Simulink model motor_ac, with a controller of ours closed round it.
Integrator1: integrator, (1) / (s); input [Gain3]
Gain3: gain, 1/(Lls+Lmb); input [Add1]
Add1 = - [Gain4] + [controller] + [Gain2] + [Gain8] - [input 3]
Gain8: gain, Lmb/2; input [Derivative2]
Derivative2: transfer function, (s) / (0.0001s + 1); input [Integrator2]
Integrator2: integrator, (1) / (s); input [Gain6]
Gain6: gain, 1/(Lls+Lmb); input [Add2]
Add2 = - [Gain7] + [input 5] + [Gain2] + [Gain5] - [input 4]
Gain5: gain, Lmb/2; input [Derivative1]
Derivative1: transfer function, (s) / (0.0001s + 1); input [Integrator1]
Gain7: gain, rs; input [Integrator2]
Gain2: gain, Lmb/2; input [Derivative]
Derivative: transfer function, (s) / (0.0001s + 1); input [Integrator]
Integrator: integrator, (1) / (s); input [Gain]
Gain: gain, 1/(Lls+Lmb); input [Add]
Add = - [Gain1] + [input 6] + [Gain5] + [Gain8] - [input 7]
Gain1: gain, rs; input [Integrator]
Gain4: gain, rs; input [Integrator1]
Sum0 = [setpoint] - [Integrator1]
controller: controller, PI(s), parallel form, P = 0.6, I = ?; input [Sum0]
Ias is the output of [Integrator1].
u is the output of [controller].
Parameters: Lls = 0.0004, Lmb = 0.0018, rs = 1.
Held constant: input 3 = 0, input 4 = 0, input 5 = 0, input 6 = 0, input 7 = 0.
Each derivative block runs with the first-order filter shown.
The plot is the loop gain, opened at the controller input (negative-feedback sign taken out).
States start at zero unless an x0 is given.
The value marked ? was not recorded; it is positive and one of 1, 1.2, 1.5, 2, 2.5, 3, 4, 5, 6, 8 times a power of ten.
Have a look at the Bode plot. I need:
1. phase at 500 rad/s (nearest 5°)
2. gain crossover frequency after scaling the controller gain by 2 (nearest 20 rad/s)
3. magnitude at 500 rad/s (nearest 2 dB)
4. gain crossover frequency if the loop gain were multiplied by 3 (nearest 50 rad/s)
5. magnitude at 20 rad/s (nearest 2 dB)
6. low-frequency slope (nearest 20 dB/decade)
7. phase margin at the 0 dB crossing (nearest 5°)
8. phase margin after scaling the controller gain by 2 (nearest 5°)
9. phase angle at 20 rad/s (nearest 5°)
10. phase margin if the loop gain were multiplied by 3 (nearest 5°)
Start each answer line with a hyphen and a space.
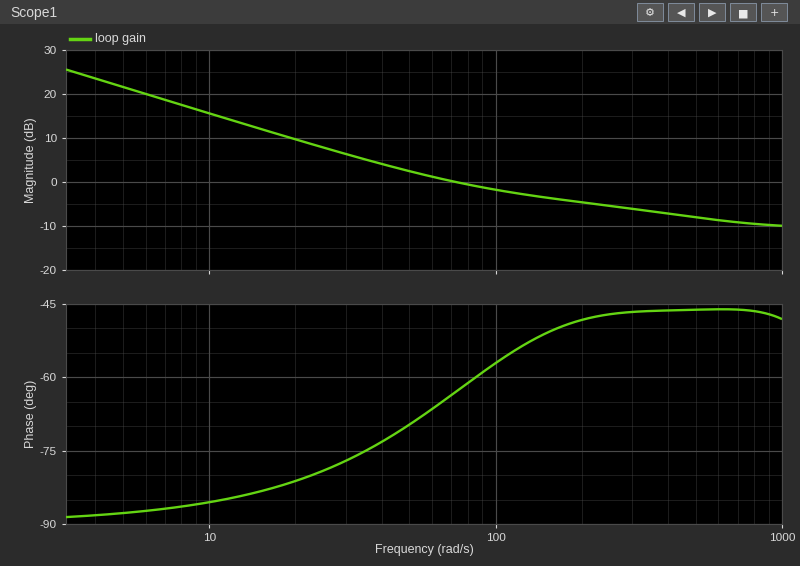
- -45°
- 300 rad/s
- -8 dB
- 800 rad/s
- 10 dB
- -20 dB/decade
- 115°
- 135°
- -80°
- 135°
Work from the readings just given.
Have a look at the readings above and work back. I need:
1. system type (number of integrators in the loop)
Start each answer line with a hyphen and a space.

- 1
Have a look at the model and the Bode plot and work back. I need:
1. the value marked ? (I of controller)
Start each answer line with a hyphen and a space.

- 60
